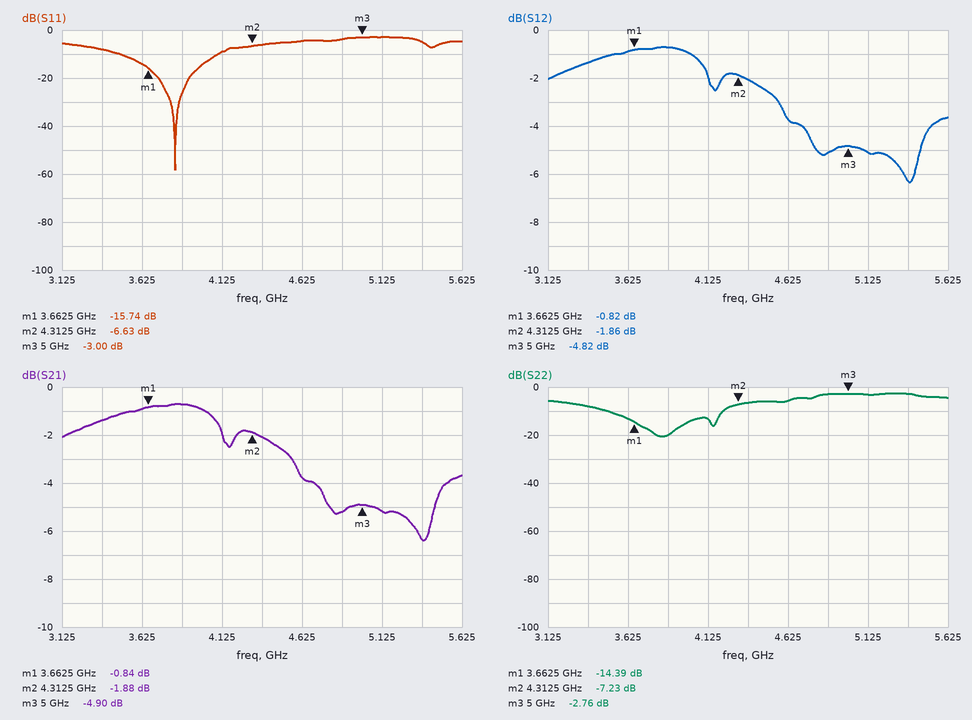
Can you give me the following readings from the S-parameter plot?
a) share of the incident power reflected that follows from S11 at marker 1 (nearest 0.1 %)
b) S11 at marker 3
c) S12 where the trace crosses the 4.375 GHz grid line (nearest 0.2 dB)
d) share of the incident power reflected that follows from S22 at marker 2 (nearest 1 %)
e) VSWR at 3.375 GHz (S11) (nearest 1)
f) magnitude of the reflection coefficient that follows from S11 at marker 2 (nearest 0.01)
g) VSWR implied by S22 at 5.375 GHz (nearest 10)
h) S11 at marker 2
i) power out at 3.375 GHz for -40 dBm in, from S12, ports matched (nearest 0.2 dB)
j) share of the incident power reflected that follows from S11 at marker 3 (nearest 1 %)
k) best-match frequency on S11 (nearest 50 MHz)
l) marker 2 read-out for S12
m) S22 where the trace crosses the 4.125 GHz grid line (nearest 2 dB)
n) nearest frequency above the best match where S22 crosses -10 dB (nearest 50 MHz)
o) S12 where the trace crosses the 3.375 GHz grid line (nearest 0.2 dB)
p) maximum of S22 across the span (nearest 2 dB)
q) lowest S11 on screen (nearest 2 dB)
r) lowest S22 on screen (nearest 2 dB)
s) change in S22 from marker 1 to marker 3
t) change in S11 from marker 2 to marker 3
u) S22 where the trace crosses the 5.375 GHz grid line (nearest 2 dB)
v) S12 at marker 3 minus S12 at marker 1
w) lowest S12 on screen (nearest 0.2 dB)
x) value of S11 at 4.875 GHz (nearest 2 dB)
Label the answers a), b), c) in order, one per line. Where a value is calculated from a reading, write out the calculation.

a) 10^(-15.74/10) ≈ 2.7 %
b) -3.00 dB
c) -2.0 dB
d) 10^(-7.23/10) ≈ 19 %
e) |Γ| = 10^(-8/20) = 0.3981; VSWR = (1 + 0.3981)/(1 − 0.3981) ≈ 2
f) 10^(-6.63/20) ≈ 0.47
g) |Γ| = 10^(-2/20) = 0.7943; VSWR = (1 + 0.7943)/(1 − 0.7943) ≈ 8.72, so 10 to the nearest 10
h) -6.63 dB
i) -40 dBm + (-1.4 dB) = -41.4 dBm
j) 10^(-3/10) ≈ 50 %
k) 3.85 GHz
l) -1.86 dB
m) -14 dB
n) 4.20 GHz
o) -1.4 dB
p) -2 dB
q) -58 dB
r) -20 dB
s) -2.76 − (-14.39) = 11.63 dB
t) -3 − (-6.63) = 3.63 dB
u) -2 dB
v) -4.82 − (-0.82) = -4.00 dB
w) -6.4 dB
x) -4 dB
